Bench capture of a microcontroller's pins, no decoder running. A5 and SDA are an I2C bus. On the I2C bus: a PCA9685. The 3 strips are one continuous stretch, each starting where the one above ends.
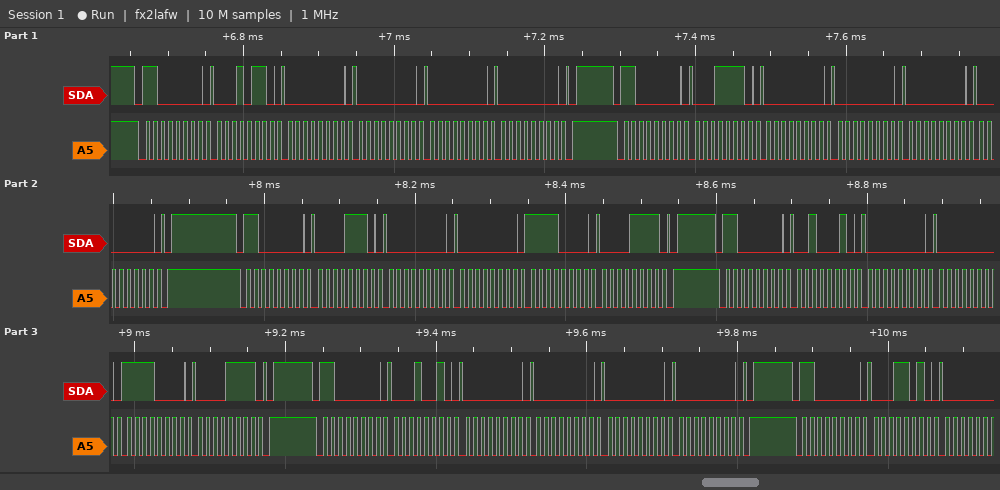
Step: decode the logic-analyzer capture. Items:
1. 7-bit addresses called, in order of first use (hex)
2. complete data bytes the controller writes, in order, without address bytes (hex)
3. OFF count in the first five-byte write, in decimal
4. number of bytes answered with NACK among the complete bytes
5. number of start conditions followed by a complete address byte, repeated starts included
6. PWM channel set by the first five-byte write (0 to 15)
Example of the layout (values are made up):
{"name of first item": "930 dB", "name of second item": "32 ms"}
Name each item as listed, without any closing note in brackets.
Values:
{"7-bit addresses called, in order of first use": "0x60", "complete data bytes the controller writes, in order, without address bytes": "16 00 00 00 00 1E 00 00 00 00 0E 00 00 F0 0F 22 00 00 F0 0F 12 00 00 00 00 1A", "OFF count in the first five-byte write, in decimal": "0", "number of bytes answered with NACK among the complete bytes": "0", "number of start conditions followed by a complete address byte, repeated starts included": "6", "PWM channel set by the first five-byte write": "4"}
